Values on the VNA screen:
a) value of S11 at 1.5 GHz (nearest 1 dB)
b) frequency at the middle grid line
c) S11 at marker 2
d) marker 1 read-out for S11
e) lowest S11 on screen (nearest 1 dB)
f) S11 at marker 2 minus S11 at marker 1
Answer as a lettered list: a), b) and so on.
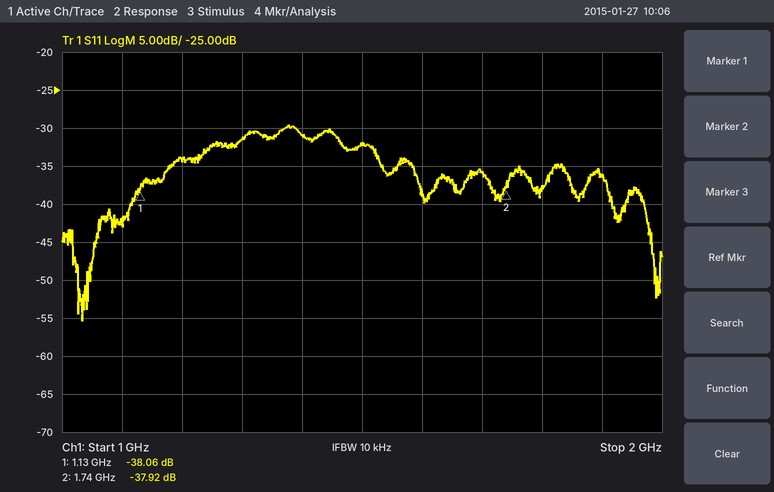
a) -32 dB
b) 1.5 GHz
c) -37.92 dB
d) -38.06 dB
e) -55 dB
f) 0.14 dB
